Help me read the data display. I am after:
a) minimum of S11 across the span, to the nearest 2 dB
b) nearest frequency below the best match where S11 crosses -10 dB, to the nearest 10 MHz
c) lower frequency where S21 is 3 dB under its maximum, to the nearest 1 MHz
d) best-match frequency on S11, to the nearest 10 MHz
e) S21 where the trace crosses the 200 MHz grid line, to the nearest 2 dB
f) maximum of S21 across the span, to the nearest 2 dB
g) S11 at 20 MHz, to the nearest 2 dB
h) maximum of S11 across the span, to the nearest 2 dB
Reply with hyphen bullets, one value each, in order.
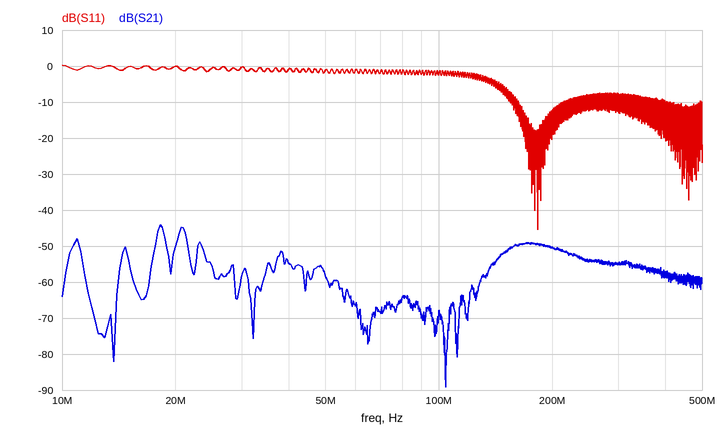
- -46 dB
- 160 MHz
- 18 MHz
- 180 MHz
- -50 dB
- -44 dB
- 0 dB
- 0 dB
